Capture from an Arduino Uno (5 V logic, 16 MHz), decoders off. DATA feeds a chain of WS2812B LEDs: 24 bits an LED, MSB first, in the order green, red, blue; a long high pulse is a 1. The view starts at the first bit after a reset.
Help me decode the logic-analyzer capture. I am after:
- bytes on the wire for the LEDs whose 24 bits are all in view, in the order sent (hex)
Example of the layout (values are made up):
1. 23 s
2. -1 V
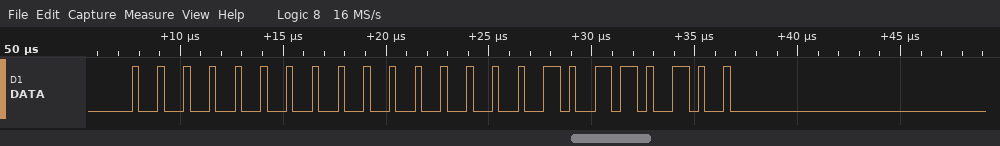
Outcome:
1. 00 00 B4
